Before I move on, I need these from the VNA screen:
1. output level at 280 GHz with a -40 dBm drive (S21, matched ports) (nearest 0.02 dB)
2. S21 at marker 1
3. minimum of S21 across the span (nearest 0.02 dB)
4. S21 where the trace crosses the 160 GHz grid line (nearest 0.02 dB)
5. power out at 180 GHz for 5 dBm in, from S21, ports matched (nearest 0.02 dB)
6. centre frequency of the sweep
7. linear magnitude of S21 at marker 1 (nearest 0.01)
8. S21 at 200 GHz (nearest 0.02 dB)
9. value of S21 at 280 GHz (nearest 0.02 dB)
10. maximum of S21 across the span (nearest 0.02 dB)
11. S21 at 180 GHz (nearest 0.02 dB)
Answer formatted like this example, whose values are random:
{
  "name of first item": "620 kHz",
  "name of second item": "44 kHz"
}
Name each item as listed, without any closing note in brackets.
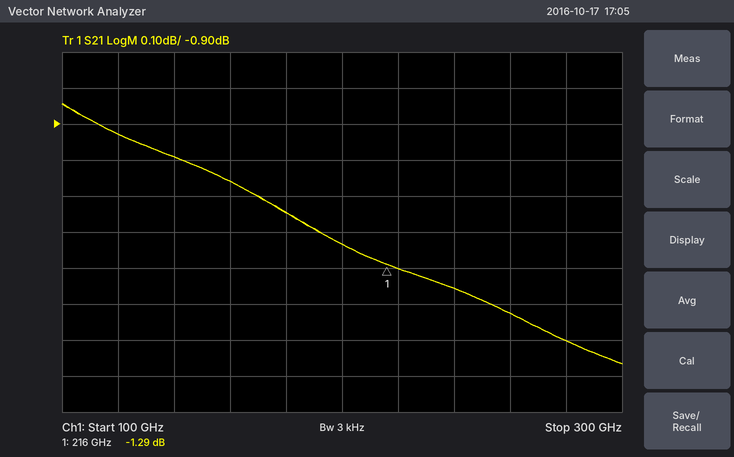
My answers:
{
  "output level at 280 GHz with a -40 dBm drive (S21, matched ports)": "-41.50 dBm",
  "S21 at marker 1": "-1.29 dB",
  "minimum of S21 across the span": "-1.56 dB",
  "S21 where the trace crosses the 160 GHz grid line": "-1.06 dB",
  "power out at 180 GHz for 5 dBm in, from S21, ports matched": "3.86 dBm",
  "centre frequency of the sweep": "200 GHz",
  "linear magnitude of S21 at marker 1": "0.86",
  "S21 at 200 GHz": "-1.24 dB",
  "value of S21 at 280 GHz": "-1.50 dB",
  "maximum of S21 across the span": "-0.84 dB",
  "S21 at 180 GHz": "-1.14 dB"
}
